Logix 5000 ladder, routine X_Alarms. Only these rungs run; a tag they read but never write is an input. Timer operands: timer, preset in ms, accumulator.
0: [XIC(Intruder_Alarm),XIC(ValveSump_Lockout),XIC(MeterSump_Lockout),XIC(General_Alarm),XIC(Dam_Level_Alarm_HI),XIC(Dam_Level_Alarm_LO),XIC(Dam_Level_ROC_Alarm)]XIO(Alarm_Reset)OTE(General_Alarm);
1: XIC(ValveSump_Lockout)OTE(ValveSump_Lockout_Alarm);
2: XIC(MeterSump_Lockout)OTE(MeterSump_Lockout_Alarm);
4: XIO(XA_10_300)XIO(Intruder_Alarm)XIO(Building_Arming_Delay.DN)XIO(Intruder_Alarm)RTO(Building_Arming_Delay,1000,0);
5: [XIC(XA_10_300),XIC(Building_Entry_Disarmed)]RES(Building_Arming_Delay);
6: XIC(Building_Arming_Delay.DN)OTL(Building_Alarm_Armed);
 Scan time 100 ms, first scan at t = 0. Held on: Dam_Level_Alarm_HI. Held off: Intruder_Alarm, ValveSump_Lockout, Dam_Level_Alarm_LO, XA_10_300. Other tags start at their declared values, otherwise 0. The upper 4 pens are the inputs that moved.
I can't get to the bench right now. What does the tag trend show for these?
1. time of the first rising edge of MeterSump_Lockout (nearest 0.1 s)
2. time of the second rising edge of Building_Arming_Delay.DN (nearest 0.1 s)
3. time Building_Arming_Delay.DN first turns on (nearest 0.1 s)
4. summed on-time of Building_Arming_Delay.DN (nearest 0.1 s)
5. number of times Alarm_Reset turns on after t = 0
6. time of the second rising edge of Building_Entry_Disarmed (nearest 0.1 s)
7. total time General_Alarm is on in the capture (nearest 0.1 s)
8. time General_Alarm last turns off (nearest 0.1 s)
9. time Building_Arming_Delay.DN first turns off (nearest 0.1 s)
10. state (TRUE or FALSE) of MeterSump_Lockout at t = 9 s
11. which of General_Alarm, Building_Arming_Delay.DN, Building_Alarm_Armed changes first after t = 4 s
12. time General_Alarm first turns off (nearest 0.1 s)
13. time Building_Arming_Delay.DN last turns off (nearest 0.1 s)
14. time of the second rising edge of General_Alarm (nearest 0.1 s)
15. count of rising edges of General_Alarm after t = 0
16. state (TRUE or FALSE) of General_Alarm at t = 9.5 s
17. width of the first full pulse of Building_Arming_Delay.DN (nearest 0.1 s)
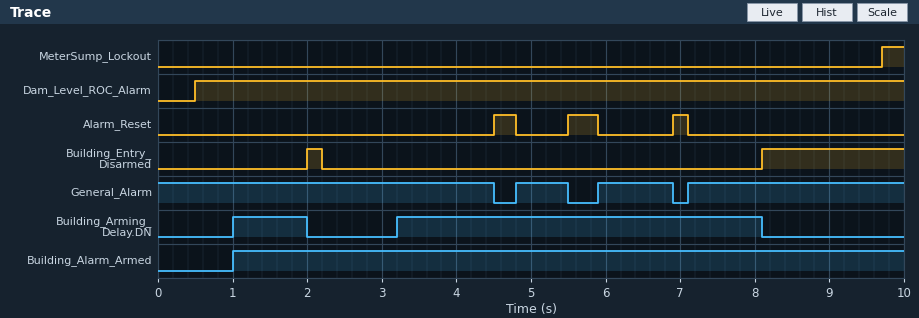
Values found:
9.7 s
3.2 s
1.0 s
5.9 s
3
8.1 s
9.1 s
6.9 s
2.0 s
FALSE
General_Alarm
4.5 s
8.1 s
5.9 s
3
TRUE
1.0 s
